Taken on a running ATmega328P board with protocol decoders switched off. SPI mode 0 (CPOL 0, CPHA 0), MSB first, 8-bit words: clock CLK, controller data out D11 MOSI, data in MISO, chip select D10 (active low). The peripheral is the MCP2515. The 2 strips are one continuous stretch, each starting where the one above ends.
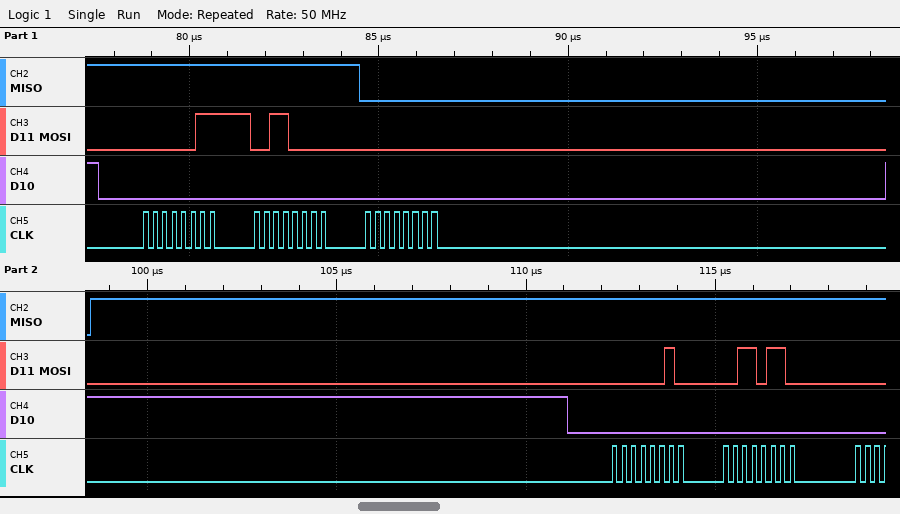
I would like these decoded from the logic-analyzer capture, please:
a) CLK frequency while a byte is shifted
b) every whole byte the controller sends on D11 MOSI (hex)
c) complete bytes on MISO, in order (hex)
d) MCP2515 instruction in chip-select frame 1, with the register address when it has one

4 MHz
0x03 0x30 0x00 0x02 0x36
0xFF 0xFF 0x00 0xFF 0xFF
READ 0x30
